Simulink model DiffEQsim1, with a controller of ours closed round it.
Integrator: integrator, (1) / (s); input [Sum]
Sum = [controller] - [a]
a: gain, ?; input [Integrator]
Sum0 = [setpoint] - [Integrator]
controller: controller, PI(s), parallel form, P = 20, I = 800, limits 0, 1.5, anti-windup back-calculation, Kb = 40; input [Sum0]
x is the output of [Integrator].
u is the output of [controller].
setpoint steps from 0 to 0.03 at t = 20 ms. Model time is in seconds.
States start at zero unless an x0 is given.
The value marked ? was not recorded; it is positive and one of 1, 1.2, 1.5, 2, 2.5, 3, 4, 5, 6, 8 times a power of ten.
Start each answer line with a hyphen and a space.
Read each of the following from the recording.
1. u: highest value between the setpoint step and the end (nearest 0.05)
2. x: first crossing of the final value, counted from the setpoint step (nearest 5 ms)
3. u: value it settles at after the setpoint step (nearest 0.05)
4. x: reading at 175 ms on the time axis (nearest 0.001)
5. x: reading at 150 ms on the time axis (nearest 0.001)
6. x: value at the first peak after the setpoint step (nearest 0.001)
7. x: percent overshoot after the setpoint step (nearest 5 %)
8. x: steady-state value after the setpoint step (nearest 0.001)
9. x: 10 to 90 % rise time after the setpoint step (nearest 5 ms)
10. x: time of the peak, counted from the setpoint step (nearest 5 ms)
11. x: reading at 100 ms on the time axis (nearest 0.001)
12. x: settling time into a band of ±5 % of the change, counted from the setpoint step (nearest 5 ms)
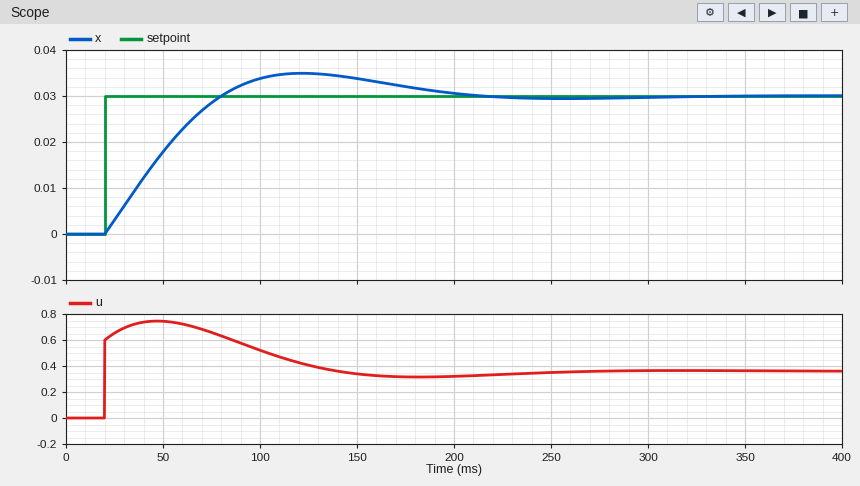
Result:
- 0.75
- 60 ms
- 0.35
- 0.032
- 0.034
- 0.035
- 15 %
- 0.030
- 45 ms
- 100 ms
- 0.034
- 165 ms
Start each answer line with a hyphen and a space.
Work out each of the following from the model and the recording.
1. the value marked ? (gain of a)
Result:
- 12
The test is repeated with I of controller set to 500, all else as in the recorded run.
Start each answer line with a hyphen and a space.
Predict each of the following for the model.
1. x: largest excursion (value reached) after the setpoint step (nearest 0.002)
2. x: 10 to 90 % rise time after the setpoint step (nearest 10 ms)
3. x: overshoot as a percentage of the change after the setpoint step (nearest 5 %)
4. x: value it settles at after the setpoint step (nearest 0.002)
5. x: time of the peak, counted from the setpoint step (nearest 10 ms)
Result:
- 0.032
- 60 ms
- 10 %
- 0.030
- 130 ms
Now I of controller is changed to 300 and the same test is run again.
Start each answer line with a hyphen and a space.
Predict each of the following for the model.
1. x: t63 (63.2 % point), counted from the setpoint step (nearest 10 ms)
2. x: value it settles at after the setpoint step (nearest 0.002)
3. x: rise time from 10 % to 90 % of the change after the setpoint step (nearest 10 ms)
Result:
- 50 ms
- 0.030
- 90 ms
